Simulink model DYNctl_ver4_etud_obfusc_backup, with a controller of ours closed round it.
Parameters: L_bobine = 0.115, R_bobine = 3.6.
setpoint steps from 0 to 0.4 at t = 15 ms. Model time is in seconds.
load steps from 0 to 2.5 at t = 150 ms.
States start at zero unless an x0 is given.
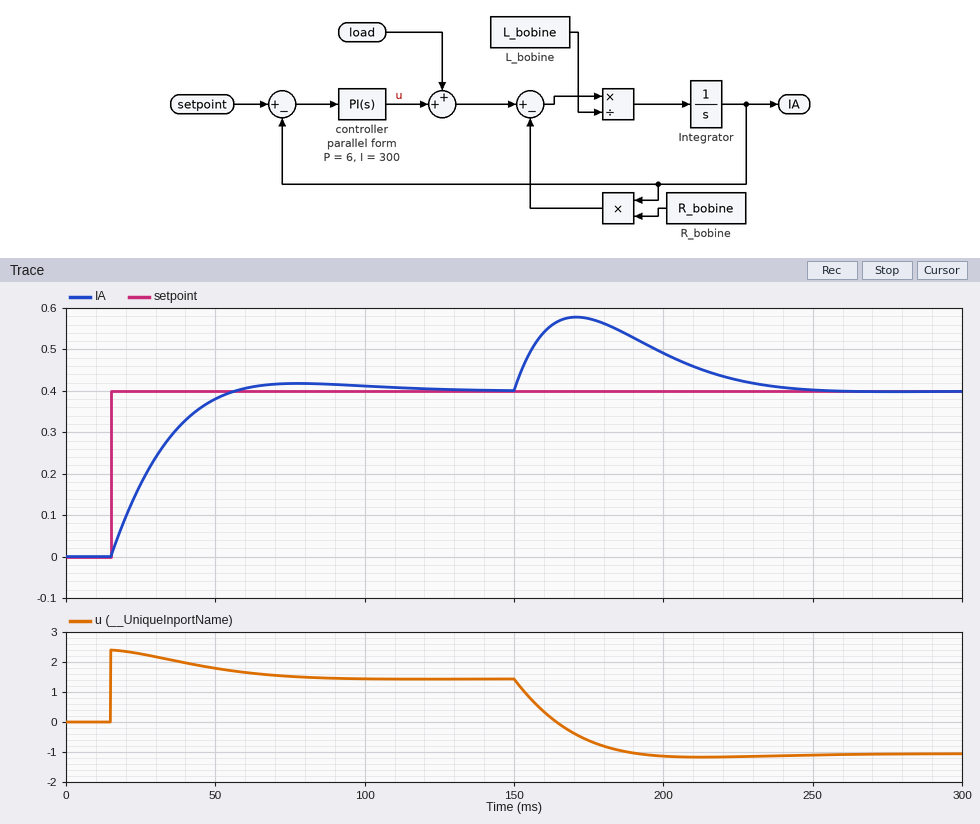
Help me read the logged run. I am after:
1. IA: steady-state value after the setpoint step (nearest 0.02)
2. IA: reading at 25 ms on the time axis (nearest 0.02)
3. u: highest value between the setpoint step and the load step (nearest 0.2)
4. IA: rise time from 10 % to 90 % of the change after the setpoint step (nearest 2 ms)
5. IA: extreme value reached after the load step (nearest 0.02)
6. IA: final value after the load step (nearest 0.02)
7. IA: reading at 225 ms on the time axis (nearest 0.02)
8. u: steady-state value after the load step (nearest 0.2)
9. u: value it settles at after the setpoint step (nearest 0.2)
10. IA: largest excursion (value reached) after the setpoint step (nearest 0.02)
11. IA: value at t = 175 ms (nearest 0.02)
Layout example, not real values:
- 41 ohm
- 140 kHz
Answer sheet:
- 0.40
- 0.18
- 2.4
- 28 ms
- 0.58
- 0.40
- 0.42
- -1.0
- 1.4
- 0.42
- 0.58
